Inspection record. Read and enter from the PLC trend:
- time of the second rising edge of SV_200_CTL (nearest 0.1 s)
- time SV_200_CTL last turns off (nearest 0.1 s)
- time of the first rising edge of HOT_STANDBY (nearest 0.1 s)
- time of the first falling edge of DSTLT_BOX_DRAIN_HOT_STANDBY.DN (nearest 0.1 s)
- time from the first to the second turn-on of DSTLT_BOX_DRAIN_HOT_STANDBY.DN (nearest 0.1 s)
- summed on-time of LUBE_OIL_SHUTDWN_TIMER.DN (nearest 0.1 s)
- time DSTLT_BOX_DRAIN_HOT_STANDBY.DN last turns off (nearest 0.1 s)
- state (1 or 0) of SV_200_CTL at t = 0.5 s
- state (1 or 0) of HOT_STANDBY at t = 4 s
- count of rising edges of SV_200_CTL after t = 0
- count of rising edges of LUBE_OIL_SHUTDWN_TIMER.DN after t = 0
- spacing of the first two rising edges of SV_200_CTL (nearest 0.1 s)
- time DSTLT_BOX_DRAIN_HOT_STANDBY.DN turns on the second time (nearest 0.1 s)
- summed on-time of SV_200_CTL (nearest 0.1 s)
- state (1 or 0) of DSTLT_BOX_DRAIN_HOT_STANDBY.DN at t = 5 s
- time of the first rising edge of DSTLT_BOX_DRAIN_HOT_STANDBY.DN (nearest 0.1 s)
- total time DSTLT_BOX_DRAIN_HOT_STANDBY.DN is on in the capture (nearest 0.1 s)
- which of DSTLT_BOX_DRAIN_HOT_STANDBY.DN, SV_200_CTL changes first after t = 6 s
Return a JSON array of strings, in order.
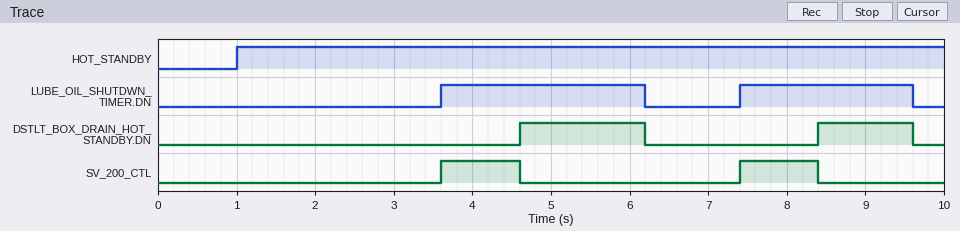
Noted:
["7.4 s", "8.4 s", "1.0 s", "6.2 s", "3.8 s", "4.8 s", "9.6 s", "0", "1", "2", "2", "3.8 s", "8.4 s", "2.0 s", "1", "4.6 s", "2.8 s", "DSTLT_BOX_DRAIN_HOT_STANDBY.DN"]
